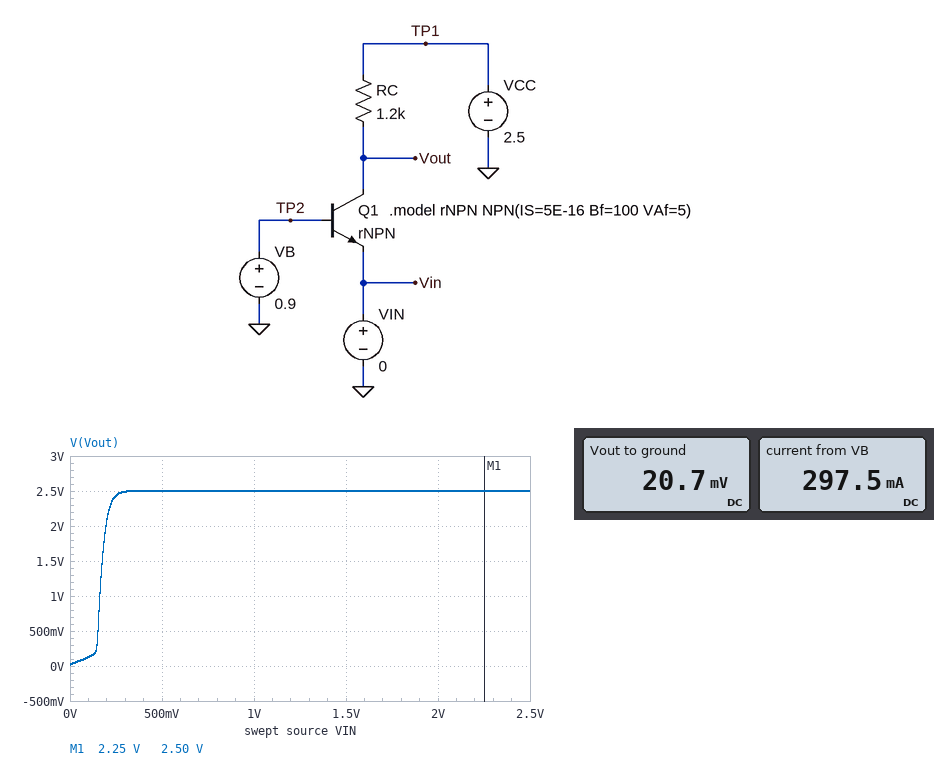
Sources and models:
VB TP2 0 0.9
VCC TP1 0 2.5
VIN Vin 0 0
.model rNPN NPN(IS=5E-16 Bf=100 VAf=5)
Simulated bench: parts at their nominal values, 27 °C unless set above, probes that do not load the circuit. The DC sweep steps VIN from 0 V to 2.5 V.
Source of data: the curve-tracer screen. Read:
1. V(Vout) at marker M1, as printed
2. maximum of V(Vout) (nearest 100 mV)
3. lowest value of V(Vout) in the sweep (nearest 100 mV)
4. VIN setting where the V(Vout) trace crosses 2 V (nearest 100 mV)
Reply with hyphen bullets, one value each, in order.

- 2.50 V
- 2.5 V
- 0 V
- 200 mV
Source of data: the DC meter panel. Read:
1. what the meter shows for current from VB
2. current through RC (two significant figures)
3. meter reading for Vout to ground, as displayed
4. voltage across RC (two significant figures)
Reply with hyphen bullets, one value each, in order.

- 297.5 mA
- 2.1 mA
- 20.7 mV
- 2.5 V
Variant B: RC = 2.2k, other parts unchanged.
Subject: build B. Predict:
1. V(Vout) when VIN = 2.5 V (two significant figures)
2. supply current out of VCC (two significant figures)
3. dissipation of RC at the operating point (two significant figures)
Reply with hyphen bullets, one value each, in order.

- 2.5 V
- 1.1 mA
- 2.8 mW
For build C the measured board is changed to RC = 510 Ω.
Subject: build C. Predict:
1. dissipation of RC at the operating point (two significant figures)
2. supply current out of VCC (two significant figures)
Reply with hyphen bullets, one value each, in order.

- 12 mW
- 4.9 mA
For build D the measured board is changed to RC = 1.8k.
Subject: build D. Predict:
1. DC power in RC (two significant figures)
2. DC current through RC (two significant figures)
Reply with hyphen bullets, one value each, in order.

- 3.4 mW
- 1.4 mA
